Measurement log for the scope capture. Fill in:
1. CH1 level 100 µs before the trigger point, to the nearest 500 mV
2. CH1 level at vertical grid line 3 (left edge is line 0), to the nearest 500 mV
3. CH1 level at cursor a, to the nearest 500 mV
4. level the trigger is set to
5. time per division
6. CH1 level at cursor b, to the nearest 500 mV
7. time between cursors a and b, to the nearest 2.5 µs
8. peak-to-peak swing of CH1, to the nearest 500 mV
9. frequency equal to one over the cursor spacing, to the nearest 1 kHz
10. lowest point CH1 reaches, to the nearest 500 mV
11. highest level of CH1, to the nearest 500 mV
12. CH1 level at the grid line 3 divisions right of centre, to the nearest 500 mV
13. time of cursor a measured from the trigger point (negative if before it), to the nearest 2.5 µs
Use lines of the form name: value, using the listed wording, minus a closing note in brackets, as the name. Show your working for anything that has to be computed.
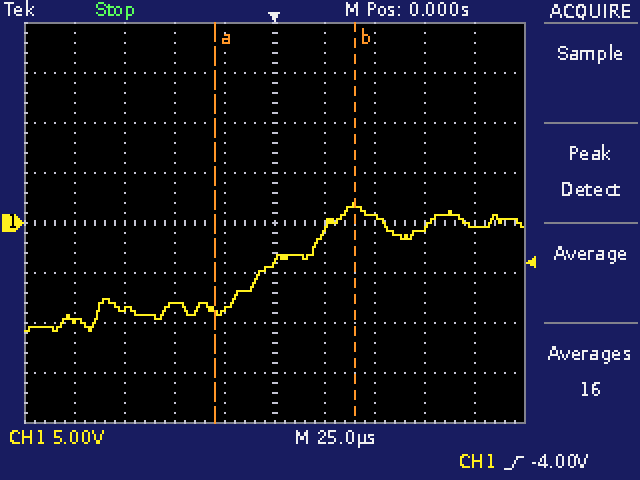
CH1 level 100 µs before the trigger point, to the nearest 500 mV: -10.0 V
CH1 level at vertical grid line 3 (left edge is line 0), to the nearest 500 mV: -8.0 V
CH1 level at cursor a, to the nearest 500 mV: -9.0 V
level the trigger is set to: -4.00 V
time per division: 25 µs
CH1 level at cursor b, to the nearest 500 mV: 1.5 V
time between cursors a and b, to the nearest 2.5 µs: 70.0 µs
peak-to-peak swing of CH1, to the nearest 500 mV: 2.0 V − (-11.0 V) = 13.0 V
frequency equal to one over the cursor spacing, to the nearest 1 kHz: 1 / 70.0 µs ≈ 14 kHz
lowest point CH1 reaches, to the nearest 500 mV: -11.0 V
highest level of CH1, to the nearest 500 mV: 2.0 V
CH1 level at the grid line 3 divisions right of centre, to the nearest 500 mV: -500 mV
time of cursor a measured from the trigger point (negative if before it), to the nearest 2.5 µs: -30.0 µs
